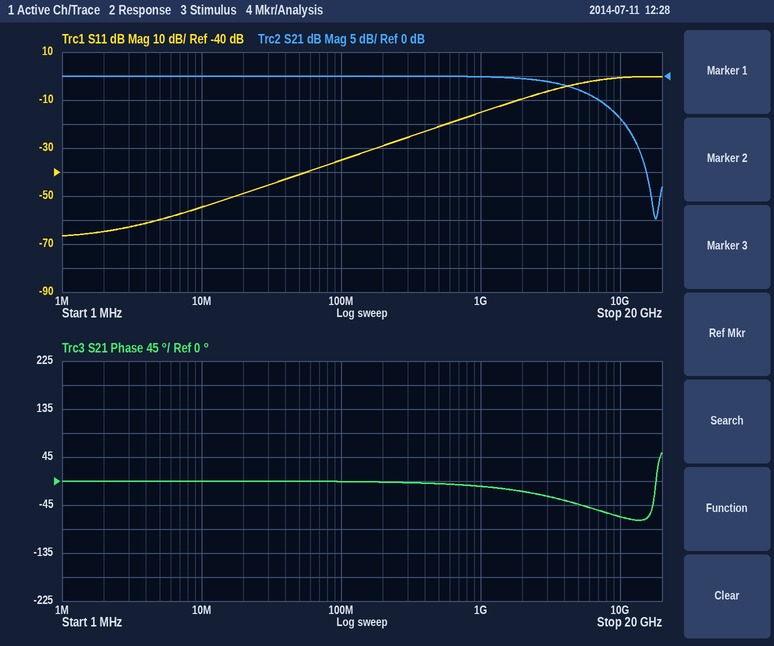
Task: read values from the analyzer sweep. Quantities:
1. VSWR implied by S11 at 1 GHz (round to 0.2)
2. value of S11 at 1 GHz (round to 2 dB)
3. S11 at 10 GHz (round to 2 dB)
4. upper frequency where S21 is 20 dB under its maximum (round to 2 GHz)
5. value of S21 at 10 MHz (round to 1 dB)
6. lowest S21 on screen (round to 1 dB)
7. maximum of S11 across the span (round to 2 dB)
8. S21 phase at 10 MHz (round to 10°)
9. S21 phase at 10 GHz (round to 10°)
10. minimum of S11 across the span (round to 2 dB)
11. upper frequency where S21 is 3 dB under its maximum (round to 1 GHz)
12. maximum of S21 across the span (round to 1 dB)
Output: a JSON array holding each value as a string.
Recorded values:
["1.4", "-16 dB", "0 dB", "16 GHz", "0 dB", "-30 dB", "0 dB", "0°", "-70°", "-66 dB", "5 GHz", "0 dB"]
